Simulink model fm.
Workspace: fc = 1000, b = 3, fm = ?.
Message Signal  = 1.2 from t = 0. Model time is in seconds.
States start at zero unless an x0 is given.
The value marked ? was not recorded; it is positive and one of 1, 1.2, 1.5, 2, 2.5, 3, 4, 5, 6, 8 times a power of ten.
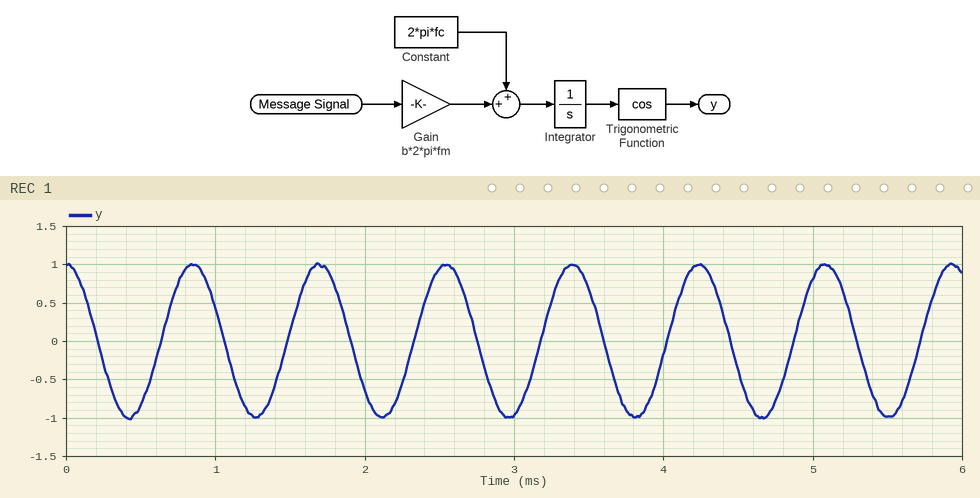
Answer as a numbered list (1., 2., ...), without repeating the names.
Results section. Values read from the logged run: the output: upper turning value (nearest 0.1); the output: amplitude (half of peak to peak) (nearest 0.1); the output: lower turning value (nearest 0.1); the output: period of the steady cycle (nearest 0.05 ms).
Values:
1. 1.0
2. 1.0
3. -1.0
4. 0.85 ms
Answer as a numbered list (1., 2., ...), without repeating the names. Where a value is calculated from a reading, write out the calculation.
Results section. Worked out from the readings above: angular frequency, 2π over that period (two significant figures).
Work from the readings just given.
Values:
1. 2π / 0.85 = 7.4 rad/ms
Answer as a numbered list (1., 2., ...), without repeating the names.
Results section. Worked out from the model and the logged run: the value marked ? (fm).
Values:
1. 50
